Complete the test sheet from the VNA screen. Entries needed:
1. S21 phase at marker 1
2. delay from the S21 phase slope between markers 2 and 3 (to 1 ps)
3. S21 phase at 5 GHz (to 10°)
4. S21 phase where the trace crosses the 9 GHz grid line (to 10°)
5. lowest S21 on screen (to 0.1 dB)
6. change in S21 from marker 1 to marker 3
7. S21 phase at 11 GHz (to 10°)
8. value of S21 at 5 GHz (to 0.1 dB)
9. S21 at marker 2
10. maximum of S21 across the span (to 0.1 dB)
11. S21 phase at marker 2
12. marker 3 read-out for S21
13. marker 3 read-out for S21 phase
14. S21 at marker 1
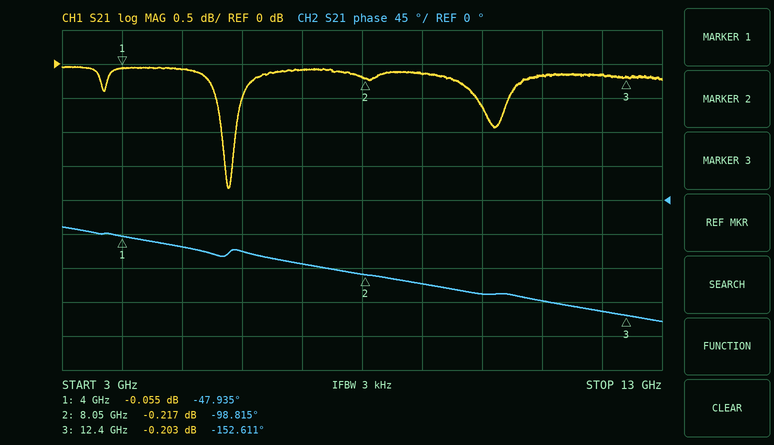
-47.935°
34 ps
-60°
-110°
-1.8 dB
-0.148 dB
-130°
-0.1 dB
-0.217 dB
0.0 dB
-98.815°
-0.203 dB
-152.611°
-0.055 dB
